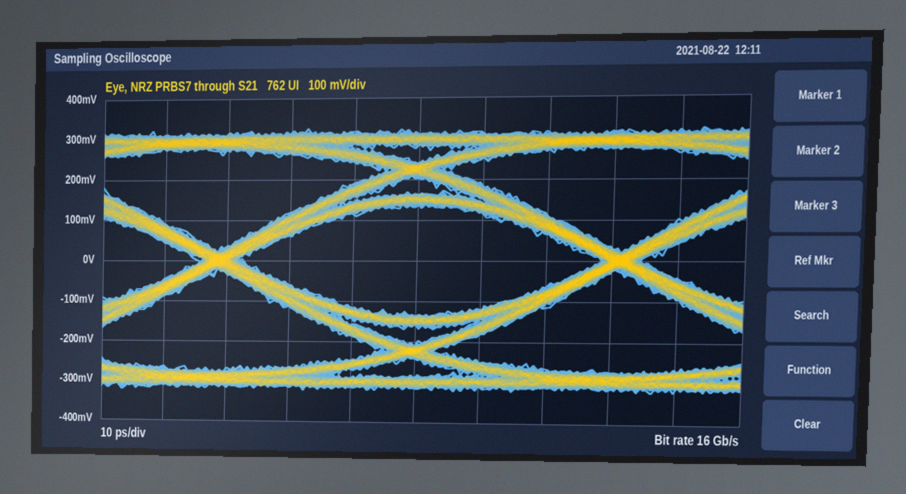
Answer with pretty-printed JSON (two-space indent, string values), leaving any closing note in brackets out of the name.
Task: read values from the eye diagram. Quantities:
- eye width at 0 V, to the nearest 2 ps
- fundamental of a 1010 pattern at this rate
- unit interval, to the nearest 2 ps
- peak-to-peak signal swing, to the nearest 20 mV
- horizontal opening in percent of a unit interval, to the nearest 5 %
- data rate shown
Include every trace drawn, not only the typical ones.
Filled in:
{
  "eye width at 0 V, to the nearest 2 ps": "56 ps",
  "fundamental of a 1010 pattern at this rate": "8 GHz",
  "unit interval, to the nearest 2 ps": "62 ps",
  "peak-to-peak signal swing, to the nearest 20 mV": "640 mV",
  "horizontal opening in percent of a unit interval, to the nearest 5 %": "90 %",
  "data rate shown": "16 Gb/s"
}
